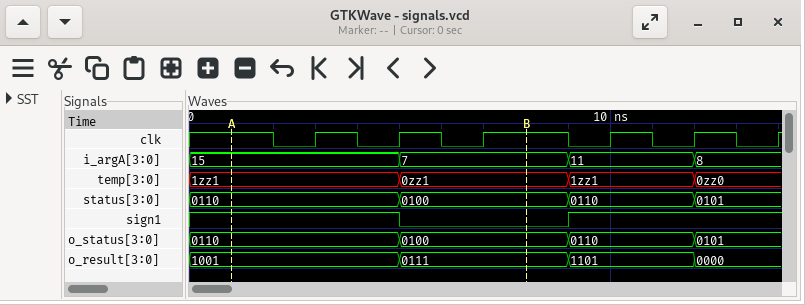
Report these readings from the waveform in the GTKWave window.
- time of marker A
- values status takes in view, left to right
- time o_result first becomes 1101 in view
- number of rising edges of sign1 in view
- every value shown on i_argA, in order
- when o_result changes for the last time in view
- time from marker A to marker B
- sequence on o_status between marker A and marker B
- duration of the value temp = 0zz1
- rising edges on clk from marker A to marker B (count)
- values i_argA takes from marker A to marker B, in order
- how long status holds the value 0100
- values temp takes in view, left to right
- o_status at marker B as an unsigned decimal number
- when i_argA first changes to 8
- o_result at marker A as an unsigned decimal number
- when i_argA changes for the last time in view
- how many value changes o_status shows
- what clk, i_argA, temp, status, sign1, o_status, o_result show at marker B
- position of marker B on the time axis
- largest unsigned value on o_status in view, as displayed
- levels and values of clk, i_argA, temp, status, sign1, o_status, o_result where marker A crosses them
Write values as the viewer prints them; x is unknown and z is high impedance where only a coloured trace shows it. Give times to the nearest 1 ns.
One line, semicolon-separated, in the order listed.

1 ns; 0110, 0100, 0110, 0101; 9 ns; 1; 15, 7, 11, 8; 12 ns; 7 ns; 0110, 0100; 4 ns; 3; 15, 7; 4 ns; 1zz1, 0zz1, 1zz1, 0zz0; 4; 12 ns; 9; 12 ns; 3; clk=1, i_argA=7, temp=0zz1, status=0100, sign1=0, o_status=0100, o_result=0111; 8 ns; 0110; clk=1, i_argA=15, temp=1zz1, status=0110, sign1=1, o_status=0110, o_result=1001
